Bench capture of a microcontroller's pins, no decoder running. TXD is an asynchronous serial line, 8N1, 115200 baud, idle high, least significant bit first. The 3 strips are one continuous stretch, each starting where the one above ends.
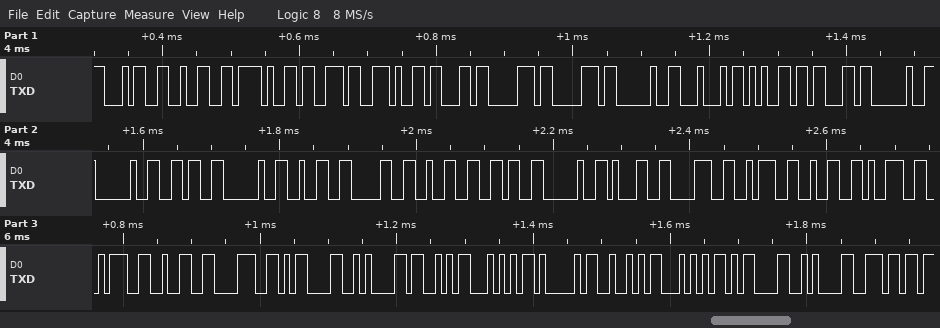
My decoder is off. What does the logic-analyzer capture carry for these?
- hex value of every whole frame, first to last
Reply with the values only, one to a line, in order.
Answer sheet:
34 32 2F 73 2E 63 70 70 20 44 65 63 20 20 36 20 32 30 32 36 20 31 38 3A 32 39 3A 32 38 0D 0A 53 54 41 52 54 0D 0A 6E
